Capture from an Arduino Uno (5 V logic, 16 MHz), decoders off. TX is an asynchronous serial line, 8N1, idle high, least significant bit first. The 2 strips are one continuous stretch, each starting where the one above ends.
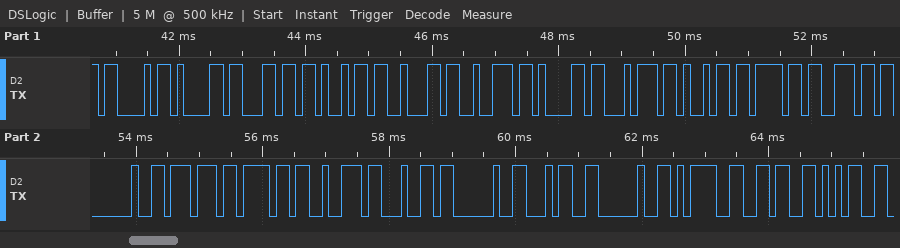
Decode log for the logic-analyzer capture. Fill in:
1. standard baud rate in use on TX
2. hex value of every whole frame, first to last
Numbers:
9600 baud
43 61 6C 69 62 72 61 74 69 6F 6E 20 77 6F 72 64 20 34 20 3D 36 35
